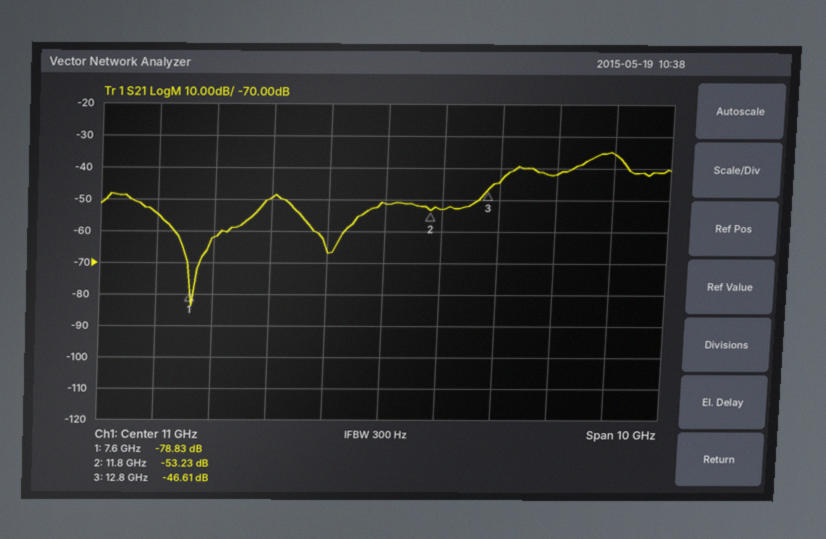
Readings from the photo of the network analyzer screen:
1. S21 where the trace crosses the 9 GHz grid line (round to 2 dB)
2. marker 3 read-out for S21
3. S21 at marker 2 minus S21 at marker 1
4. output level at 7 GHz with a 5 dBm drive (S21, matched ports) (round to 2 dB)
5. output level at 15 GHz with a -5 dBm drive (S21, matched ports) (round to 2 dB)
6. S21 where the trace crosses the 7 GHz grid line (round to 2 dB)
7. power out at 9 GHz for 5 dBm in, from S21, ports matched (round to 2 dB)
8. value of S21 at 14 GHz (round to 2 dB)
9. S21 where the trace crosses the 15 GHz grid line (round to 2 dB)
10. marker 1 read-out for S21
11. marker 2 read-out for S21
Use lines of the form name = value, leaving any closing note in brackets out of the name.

S21 where the trace crosses the 9 GHz grid line = -50 dB
marker 3 read-out for S21 = -46.61 dB
S21 at marker 2 minus S21 at marker 1 = 25.60 dB
output level at 7 GHz with a 5 dBm drive (S21, matched ports) = -50 dBm
output level at 15 GHz with a -5 dBm drive (S21, matched ports) = -40 dBm
S21 where the trace crosses the 7 GHz grid line = -54 dB
power out at 9 GHz for 5 dBm in, from S21, ports matched = -44 dBm
value of S21 at 14 GHz = -42 dB
S21 where the trace crosses the 15 GHz grid line = -36 dB
marker 1 read-out for S21 = -78.83 dB
marker 2 read-out for S21 = -53.23 dB
